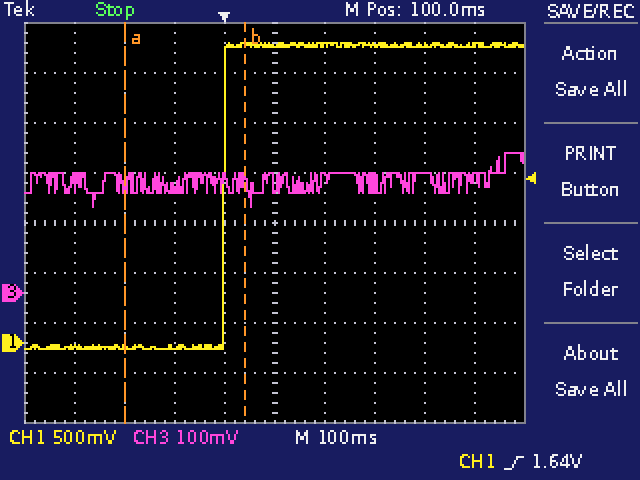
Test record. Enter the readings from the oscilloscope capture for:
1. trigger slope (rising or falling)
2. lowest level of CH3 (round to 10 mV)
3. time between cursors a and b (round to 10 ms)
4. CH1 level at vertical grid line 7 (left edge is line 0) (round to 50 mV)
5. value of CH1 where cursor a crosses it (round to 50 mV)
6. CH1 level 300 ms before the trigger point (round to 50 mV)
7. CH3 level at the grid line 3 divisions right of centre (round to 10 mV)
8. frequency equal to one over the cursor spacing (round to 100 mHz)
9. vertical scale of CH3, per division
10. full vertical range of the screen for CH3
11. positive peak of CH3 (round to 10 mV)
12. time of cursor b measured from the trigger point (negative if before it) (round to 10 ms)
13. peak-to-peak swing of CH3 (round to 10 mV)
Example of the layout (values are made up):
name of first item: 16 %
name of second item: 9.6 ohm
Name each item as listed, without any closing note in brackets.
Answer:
trigger slope: rising
lowest level of CH3: 170 mV
time between cursors a and b: 240 ms
CH1 level at vertical grid line 7 (left edge is line 0): 3.00 V
value of CH1 where cursor a crosses it: -50 mV
CH1 level 300 ms before the trigger point: -50 mV
CH3 level at the grid line 3 divisions right of centre: 240 mV
frequency equal to one over the cursor spacing: 4.2 Hz
vertical scale of CH3, per division: 100 mV
full vertical range of the screen for CH3: 800 mV
positive peak of CH3: 280 mV
time of cursor b measured from the trigger point (negative if before it): +40 ms
peak-to-peak swing of CH3: 110 mV
